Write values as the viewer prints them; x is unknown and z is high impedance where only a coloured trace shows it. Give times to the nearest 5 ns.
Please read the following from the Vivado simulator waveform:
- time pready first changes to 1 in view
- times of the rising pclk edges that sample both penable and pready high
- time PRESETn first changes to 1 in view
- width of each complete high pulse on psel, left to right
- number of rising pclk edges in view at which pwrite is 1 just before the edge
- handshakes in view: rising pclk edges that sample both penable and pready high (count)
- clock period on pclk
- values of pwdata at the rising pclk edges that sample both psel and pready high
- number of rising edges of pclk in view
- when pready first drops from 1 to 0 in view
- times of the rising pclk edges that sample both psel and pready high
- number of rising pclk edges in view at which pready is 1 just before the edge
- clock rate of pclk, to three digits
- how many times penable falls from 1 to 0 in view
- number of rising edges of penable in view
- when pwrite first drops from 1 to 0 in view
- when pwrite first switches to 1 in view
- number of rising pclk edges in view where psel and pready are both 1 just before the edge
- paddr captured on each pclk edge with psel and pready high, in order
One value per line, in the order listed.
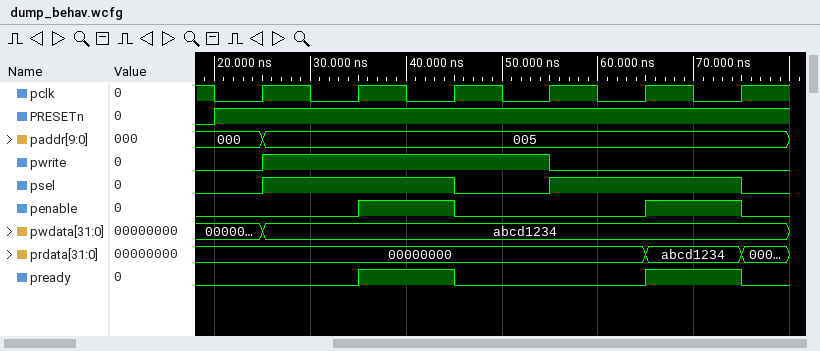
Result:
35 ns
45 ns, 75 ns
20 ns
20 ns, 20 ns
3
2
10 ns
abcd1234, abcd1234
6
45 ns
45 ns, 75 ns
2
100 MHz
2
2
55 ns
25 ns
2
005, 005
